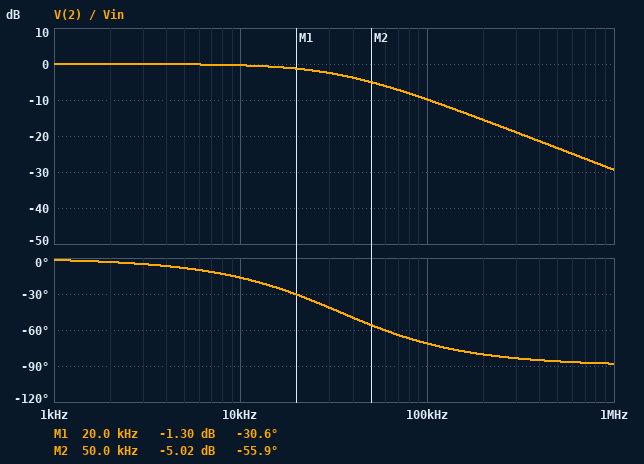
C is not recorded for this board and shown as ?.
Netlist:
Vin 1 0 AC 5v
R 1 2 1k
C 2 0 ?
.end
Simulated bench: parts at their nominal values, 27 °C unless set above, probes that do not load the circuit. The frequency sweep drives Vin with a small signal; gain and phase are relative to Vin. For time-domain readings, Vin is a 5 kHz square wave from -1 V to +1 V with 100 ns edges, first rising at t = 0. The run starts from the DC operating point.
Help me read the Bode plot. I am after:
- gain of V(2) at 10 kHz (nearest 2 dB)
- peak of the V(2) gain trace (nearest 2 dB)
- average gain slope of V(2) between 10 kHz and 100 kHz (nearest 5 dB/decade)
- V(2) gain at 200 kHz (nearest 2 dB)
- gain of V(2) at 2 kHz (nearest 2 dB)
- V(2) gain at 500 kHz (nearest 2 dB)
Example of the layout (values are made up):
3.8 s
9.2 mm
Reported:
0 dB
0 dB
-10 dB/decade
-16 dB
0 dB
-24 dB
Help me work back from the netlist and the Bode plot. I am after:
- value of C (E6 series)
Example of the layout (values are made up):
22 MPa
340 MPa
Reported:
4.7 nF
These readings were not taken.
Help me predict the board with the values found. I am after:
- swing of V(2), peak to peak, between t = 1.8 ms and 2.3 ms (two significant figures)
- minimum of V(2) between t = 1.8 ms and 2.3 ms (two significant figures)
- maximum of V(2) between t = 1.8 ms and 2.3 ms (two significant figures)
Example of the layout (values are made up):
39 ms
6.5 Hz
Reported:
2.0 V
-1.0 V
1.0 V
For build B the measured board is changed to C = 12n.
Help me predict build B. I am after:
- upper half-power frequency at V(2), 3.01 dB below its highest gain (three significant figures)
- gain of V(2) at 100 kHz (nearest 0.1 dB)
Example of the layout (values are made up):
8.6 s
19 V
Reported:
13.3 kHz
-17.6 dB
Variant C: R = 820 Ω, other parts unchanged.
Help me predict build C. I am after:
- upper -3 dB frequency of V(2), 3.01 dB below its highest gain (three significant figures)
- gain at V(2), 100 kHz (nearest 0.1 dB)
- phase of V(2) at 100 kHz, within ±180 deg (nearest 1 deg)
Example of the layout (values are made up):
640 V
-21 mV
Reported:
41.3 kHz
-8.4 dB
-68 deg
